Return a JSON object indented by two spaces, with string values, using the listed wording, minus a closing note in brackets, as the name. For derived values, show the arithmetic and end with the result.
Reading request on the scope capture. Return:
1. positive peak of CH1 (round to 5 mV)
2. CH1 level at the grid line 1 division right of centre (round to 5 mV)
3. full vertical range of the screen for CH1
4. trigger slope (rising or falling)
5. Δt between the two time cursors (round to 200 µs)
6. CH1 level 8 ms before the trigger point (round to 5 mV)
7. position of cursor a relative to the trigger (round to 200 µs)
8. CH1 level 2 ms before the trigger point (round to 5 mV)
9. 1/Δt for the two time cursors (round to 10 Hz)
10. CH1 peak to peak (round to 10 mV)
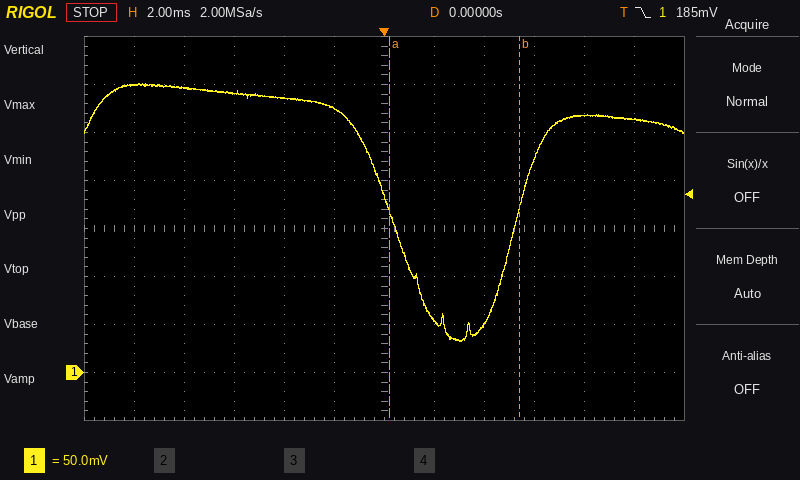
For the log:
{
  "positive peak of CH1": "300 mV",
  "CH1 level at the grid line 1 division right of centre": "55 mV",
  "full vertical range of the screen for CH1": "400 mV",
  "trigger slope": "falling",
  "Δt between the two time cursors": "5.2 ms",
  "CH1 level 8 ms before the trigger point": "295 mV",
  "position of cursor a relative to the trigger": "+200 µs",
  "CH1 level 2 ms before the trigger point": "275 mV",
  "1/Δt for the two time cursors": "1 / 5.2 ms ≈ 190 Hz",
  "CH1 peak to peak": "270 mV"
}
